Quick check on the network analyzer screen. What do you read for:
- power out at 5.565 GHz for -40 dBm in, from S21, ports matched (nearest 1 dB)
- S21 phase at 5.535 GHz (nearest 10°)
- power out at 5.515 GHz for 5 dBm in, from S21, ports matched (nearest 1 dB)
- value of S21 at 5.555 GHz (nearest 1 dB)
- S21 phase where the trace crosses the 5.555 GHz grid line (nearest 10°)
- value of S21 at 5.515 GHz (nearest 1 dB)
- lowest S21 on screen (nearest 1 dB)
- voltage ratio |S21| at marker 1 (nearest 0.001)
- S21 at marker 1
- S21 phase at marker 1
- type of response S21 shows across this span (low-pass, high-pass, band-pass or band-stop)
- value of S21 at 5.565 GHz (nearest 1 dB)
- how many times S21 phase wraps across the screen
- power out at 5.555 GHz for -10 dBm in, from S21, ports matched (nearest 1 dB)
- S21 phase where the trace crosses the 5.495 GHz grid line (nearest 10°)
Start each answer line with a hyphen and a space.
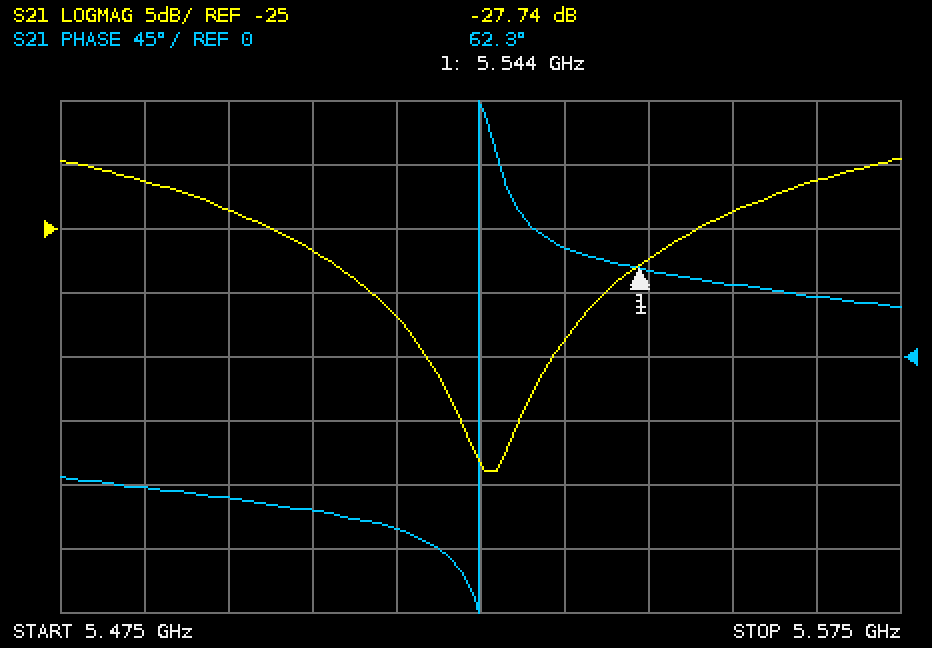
- -61 dBm
- 80°
- -27 dBm
- -24 dB
- 50°
- -32 dB
- -44 dB
- 0.041
- -27.74 dB
- 62.3°
- band-stop
- -21 dB
- 1
- -34 dBm
- -100°
